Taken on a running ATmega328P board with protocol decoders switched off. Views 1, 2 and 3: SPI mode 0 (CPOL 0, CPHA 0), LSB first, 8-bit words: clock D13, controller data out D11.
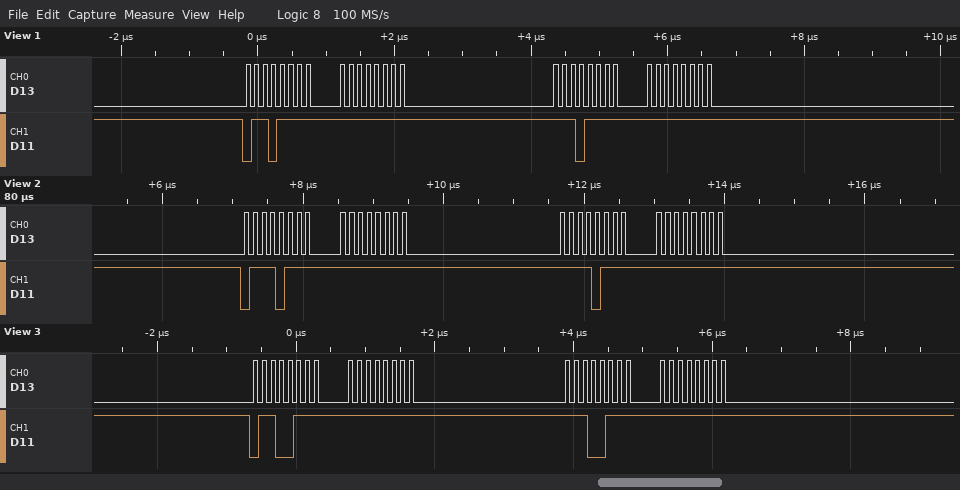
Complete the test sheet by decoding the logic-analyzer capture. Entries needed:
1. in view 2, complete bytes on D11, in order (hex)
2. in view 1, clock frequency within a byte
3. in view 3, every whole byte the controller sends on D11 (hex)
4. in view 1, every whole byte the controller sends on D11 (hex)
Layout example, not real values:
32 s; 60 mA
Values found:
EE FF EF FF; 8 MHz; E6 FF E7 FF; F6 FF F7 FF
